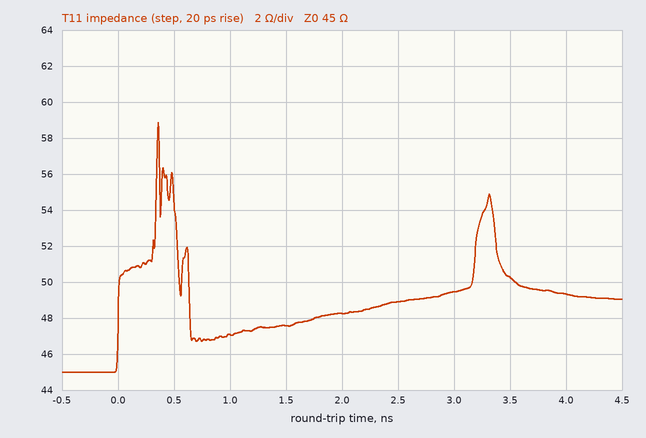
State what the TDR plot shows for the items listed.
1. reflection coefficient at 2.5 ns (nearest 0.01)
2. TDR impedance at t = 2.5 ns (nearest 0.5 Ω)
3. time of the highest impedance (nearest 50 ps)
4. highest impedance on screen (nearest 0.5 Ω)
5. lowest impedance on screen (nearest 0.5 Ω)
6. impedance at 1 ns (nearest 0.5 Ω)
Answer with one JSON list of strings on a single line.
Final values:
["+0.04", "49.0 Ω", "350 ps", "59.0 Ω", "45.0 Ω", "47.0 Ω"]
